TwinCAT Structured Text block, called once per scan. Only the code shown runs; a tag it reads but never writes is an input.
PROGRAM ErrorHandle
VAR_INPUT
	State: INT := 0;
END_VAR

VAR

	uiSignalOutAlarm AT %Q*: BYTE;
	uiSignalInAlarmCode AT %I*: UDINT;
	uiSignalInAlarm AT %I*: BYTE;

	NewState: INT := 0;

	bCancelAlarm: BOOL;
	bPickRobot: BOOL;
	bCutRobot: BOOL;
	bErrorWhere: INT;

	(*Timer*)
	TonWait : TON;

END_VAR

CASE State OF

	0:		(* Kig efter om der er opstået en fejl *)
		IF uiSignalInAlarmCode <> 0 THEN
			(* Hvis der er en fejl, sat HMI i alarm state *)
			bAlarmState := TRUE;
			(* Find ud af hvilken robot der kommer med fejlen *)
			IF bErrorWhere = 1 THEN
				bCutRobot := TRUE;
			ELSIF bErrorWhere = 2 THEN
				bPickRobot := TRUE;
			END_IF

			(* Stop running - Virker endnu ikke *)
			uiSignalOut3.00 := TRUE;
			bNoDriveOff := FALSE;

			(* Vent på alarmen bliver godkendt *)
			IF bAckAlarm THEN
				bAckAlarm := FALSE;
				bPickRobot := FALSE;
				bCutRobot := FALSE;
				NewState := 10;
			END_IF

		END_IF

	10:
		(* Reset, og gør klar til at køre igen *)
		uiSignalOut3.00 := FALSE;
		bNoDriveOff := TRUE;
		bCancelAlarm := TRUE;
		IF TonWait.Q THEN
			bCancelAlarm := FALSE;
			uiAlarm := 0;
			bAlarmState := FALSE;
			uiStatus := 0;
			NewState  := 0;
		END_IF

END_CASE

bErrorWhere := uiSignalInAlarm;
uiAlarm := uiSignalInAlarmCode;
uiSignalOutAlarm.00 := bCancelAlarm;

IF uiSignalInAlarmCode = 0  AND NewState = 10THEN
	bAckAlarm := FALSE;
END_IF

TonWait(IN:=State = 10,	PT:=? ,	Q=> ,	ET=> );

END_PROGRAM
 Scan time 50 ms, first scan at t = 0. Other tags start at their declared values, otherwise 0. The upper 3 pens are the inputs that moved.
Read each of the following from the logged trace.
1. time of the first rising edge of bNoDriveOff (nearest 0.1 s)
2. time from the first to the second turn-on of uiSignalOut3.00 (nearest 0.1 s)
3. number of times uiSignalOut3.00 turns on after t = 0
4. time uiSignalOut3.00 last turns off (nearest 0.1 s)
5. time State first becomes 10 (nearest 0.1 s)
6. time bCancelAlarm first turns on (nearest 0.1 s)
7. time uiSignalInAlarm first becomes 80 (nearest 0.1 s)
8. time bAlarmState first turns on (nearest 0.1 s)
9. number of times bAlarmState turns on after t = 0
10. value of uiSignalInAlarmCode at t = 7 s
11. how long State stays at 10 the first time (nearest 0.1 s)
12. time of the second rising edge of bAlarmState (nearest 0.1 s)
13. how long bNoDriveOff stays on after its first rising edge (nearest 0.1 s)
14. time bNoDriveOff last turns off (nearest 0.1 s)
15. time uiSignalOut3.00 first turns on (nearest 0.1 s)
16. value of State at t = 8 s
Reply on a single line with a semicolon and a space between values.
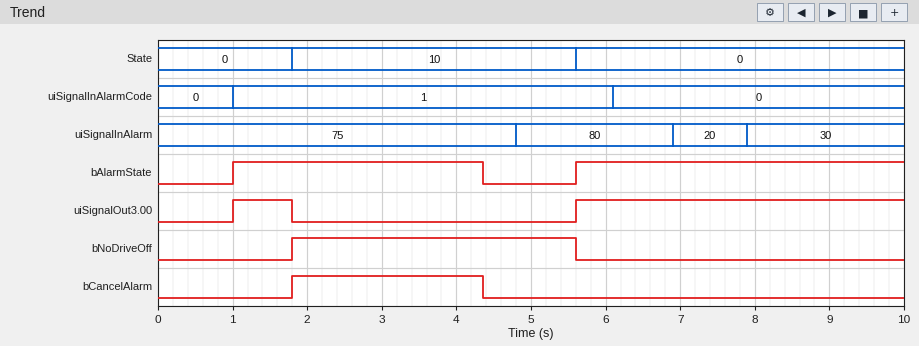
1.8 s; 4.6 s; 2; 1.8 s; 1.8 s; 1.8 s; 4.8 s; 1.0 s; 2; 0; 3.8 s; 5.6 s; 3.8 s; 5.6 s; 1.0 s; 0
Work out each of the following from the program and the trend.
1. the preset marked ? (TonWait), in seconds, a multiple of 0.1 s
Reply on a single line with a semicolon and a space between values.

2.5 s
